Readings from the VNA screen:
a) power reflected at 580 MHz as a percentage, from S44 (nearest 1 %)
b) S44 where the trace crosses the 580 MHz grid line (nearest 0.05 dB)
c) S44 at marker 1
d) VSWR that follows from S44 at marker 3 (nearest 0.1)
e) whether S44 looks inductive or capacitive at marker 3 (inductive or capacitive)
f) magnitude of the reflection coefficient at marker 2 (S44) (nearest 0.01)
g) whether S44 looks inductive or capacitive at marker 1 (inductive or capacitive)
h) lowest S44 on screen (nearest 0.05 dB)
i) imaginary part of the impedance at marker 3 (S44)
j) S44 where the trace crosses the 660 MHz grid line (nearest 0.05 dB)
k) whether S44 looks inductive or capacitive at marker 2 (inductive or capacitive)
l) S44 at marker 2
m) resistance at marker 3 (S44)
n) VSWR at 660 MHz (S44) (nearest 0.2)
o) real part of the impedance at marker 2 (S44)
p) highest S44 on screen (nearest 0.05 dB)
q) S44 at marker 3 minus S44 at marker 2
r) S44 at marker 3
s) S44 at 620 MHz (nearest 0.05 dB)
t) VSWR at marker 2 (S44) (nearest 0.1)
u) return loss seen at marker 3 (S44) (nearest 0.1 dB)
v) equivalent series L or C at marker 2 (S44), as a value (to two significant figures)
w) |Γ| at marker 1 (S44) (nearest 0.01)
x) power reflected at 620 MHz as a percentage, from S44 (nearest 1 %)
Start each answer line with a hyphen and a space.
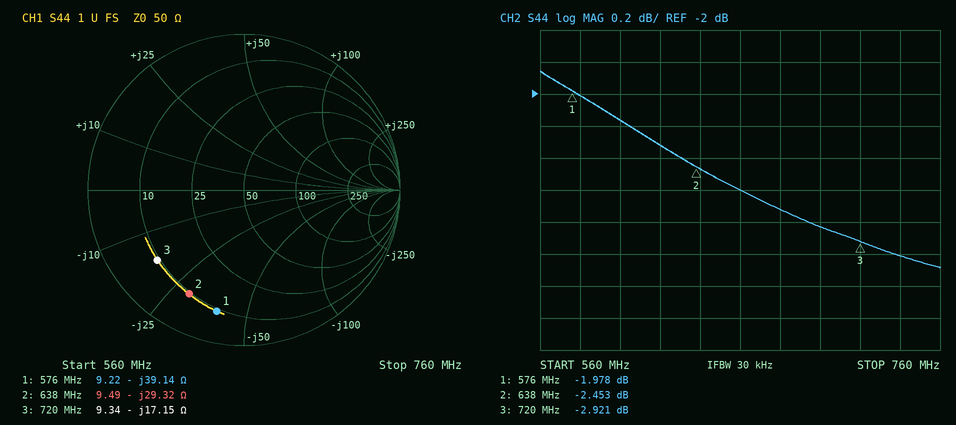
- 63 %
- -2.00 dB
- -1.978 dB
- 6.0
- capacitive
- 0.75
- capacitive
- -3.10 dB
- -17.15 Ω
- -2.60 dB
- capacitive
- -2.453 dB
- 9.34 Ω
- 6.8
- 9.49 Ω
- -1.85 dB
- -0.468 dB
- -2.921 dB
- -2.30 dB
- 7.1
- 2.9 dB
- 8.5 pF
- 0.80
- 59 %
